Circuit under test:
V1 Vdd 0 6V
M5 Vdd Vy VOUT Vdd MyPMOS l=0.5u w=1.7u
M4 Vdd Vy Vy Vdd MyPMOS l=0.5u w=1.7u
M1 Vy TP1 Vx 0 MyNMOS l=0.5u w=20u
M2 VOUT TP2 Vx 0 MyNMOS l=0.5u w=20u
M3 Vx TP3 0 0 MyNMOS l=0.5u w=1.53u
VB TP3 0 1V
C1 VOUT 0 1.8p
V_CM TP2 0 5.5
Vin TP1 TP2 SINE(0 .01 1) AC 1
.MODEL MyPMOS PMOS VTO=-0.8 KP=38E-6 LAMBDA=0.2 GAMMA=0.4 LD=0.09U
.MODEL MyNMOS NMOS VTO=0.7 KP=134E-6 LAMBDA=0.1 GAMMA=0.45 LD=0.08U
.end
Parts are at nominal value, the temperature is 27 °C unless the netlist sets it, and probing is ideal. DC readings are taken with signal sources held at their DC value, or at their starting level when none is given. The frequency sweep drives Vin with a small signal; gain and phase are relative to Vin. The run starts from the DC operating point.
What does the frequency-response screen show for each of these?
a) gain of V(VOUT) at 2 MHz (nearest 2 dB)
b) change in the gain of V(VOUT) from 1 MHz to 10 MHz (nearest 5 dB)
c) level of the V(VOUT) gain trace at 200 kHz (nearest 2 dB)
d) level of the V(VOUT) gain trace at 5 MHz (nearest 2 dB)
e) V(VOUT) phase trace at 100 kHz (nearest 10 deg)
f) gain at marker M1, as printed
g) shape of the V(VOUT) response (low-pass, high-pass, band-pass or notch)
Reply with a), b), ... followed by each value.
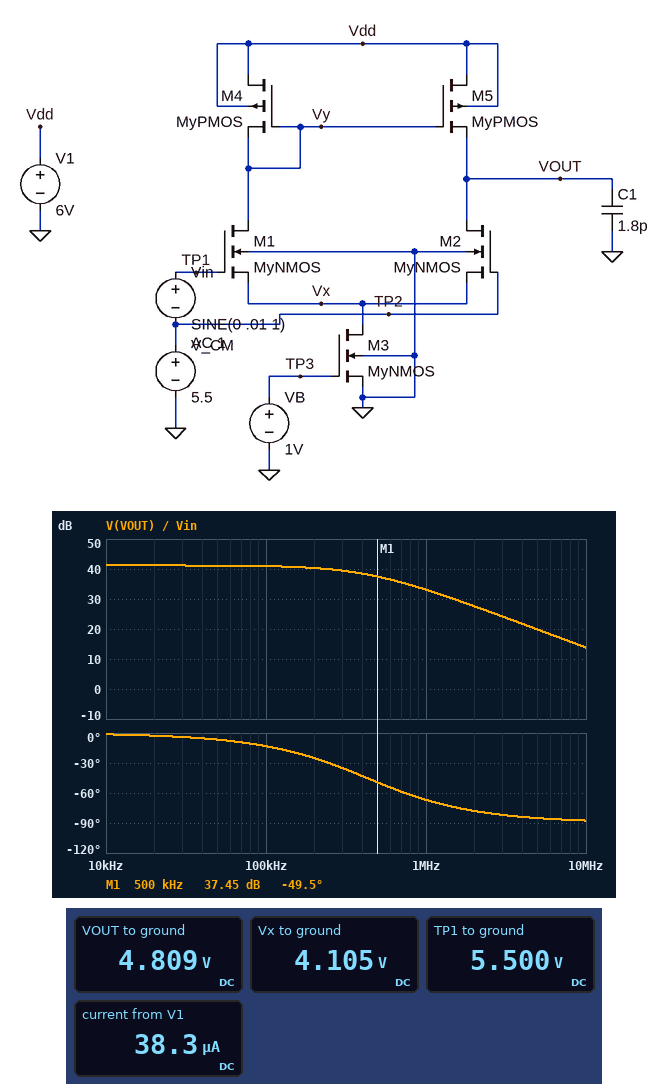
a) 28 dB
b) -20 dB
c) 40 dB
d) 20 dB
e) -10 deg
f) 37.45 dB
g) low-pass
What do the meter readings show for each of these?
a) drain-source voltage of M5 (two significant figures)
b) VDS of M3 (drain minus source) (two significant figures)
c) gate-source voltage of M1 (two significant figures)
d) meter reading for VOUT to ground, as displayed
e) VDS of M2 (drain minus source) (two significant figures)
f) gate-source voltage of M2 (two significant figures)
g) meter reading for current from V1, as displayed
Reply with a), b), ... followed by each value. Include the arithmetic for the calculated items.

a) 6 V - 4.809 V = 1.2 V
b) 4.105 V = 4.1 V
c) 5.5 V - 4.105 V = 1.4 V
d) 4.809 V
e) 4.809 V - 4.105 V = 700 mV
f) 5.5 V - 4.105 V = 1.4 V
g) 38.3 µA
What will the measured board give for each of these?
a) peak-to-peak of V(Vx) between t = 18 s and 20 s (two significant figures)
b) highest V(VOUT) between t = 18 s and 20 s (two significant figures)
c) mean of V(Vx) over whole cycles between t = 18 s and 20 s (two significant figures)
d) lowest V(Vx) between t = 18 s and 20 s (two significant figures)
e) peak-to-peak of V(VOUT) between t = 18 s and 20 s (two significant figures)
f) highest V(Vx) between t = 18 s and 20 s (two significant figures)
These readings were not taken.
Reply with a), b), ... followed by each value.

a) 13 mV
b) 5.7 V
c) 4.1 V
d) 4.1 V
e) 1.5 V
f) 4.1 V
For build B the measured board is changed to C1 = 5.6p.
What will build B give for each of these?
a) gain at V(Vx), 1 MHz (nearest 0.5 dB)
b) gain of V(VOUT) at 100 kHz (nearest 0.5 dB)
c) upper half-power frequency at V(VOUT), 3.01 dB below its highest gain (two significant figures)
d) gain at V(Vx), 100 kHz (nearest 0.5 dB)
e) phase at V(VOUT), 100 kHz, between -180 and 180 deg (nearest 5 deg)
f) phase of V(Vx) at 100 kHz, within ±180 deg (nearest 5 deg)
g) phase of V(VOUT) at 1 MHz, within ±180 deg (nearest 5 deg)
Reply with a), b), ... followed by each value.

a) -7.0 dB
b) 39.5 dB
c) 140 kHz
d) -5.0 dB
e) -35 deg
f) -10 deg
g) -80 deg
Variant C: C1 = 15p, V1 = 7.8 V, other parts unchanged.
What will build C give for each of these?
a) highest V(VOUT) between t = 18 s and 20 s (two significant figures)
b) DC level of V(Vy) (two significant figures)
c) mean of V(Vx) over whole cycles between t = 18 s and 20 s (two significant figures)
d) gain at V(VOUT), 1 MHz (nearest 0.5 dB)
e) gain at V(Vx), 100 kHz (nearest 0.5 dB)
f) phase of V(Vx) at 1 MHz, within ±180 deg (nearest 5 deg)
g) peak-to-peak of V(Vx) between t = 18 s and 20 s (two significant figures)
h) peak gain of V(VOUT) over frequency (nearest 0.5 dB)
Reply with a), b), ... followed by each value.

a) 7.5 V
b) 6.6 V
c) 4.1 V
d) 16.0 dB
e) -6.5 dB
f) 0 deg
g) 12 mV
h) 42.5 dB
